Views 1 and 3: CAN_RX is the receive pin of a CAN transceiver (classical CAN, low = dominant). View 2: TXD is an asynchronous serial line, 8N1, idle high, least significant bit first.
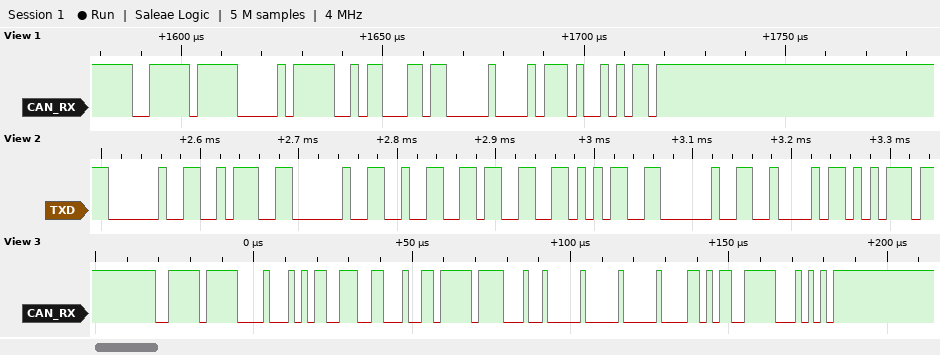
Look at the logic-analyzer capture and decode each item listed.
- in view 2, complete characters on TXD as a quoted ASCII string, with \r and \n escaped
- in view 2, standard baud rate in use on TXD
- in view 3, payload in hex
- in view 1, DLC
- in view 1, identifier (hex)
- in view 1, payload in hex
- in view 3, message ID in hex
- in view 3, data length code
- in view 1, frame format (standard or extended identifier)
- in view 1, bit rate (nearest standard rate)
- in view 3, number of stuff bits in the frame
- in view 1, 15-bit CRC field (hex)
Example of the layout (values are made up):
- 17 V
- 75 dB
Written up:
- " : 235 Bu"
- 115200 baud
- AC E6 26 FF 89 00 00 1A
- 3
- 0x3FF
- EB 1B 00
- 0x3FF
- 8
- standard
- 500 kbit/s
- 7
- 0x2E95
